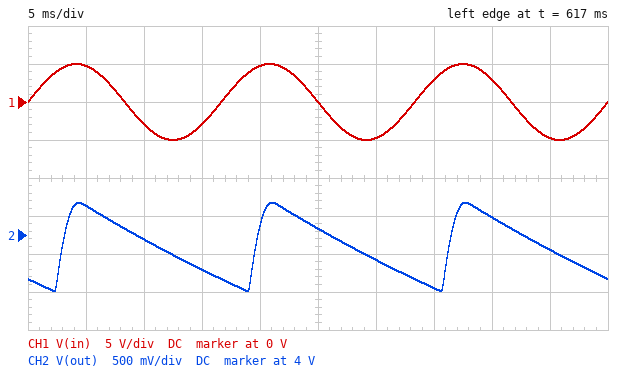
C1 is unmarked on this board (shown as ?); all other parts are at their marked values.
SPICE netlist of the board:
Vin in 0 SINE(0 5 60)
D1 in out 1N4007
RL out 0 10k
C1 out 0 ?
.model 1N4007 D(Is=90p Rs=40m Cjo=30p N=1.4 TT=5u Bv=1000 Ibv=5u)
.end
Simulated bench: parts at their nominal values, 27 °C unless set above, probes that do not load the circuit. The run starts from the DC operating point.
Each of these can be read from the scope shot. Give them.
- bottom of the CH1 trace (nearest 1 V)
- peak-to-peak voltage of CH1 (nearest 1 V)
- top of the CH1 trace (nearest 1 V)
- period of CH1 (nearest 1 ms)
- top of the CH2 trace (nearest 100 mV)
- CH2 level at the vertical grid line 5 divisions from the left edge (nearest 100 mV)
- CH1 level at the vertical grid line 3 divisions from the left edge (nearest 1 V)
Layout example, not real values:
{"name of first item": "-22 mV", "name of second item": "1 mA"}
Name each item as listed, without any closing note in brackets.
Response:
{"bottom of the CH1 trace": "-5 V", "peak-to-peak voltage of CH1": "10 V", "top of the CH1 trace": "5 V", "period of CH1": "17 ms", "top of the CH2 trace": "4.4 V", "CH2 level at the vertical grid line 5 divisions from the left edge": "4.1 V", "CH1 level at the vertical grid line 3 divisions from the left edge": "-3 V"}
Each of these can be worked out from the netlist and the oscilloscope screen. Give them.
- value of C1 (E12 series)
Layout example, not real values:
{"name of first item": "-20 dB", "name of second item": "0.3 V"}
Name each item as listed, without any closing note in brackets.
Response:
{"value of C1": "4.7 µF"}
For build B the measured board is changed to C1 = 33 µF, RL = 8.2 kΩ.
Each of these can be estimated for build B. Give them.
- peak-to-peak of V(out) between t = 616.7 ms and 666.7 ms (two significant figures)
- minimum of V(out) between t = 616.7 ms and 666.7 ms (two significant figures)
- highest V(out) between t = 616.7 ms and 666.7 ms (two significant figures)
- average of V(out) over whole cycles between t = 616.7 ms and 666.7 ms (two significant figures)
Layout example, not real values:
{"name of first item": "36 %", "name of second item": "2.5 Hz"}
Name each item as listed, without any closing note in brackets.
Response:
{"peak-to-peak of V(out) between t = 616.7 ms and 666.7 ms": "240 mV", "minimum of V(out) between t = 616.7 ms and 666.7 ms": "4.1 V", "highest V(out) between t = 616.7 ms and 666.7 ms": "4.4 V", "average of V(out) over whole cycles between t = 616.7 ms and 666.7 ms": "4.3 V"}
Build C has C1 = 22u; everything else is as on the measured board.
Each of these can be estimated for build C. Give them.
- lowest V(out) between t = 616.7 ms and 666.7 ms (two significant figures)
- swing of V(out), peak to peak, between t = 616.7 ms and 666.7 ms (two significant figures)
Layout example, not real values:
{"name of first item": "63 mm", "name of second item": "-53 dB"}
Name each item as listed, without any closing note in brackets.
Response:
{"lowest V(out) between t = 616.7 ms and 666.7 ms": "4.1 V", "swing of V(out), peak to peak, between t = 616.7 ms and 666.7 ms": "290 mV"}
